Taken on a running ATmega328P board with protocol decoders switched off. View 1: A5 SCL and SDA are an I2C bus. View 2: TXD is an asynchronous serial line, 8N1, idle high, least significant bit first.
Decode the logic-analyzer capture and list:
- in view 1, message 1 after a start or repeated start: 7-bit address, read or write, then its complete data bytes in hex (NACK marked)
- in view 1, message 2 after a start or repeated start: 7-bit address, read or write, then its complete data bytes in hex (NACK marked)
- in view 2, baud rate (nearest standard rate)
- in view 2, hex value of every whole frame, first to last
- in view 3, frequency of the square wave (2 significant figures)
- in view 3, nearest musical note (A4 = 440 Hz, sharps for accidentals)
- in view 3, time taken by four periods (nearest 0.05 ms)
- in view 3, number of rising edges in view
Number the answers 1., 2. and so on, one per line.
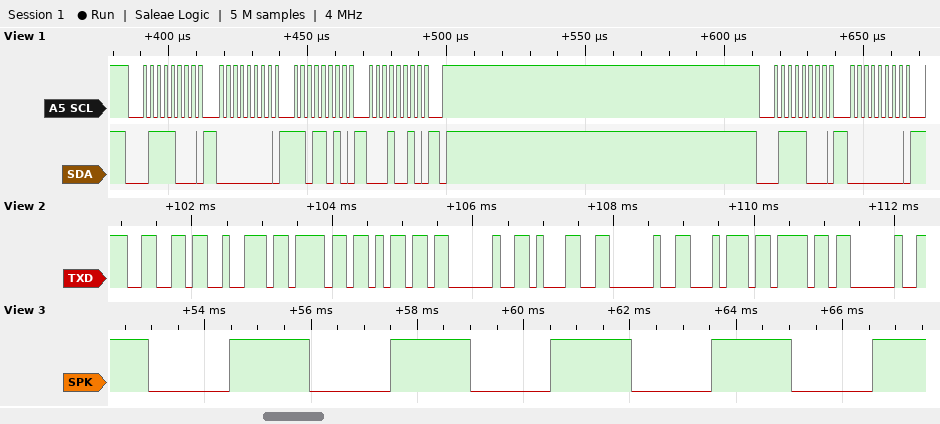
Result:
1. 0x3C write: 00 DA 12
2. 0x3C write: 00
3. 9600 baud
4. 0x66 0x72 0x6F 0x6D 0x20 0x31 0x20 0x74 0x6F 0x20
5. 330 Hz
6. E4
7. 12.10 ms
8. 5
